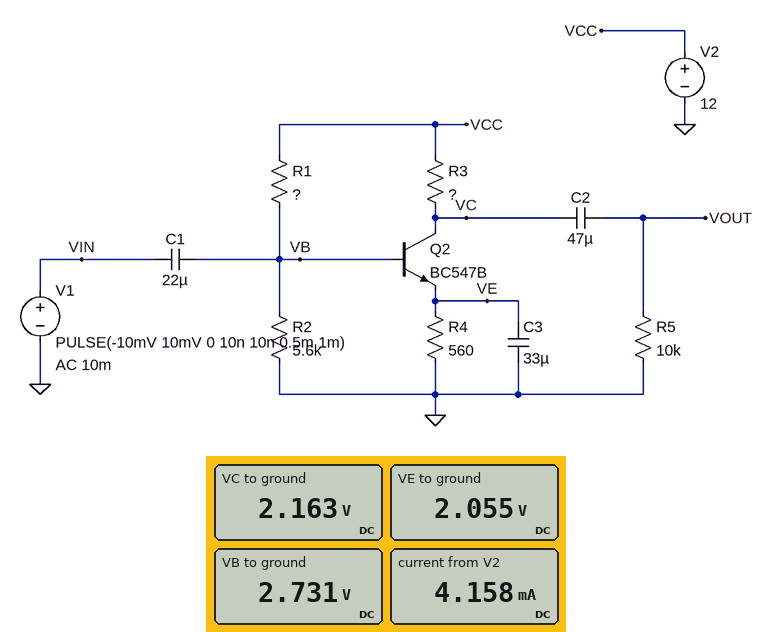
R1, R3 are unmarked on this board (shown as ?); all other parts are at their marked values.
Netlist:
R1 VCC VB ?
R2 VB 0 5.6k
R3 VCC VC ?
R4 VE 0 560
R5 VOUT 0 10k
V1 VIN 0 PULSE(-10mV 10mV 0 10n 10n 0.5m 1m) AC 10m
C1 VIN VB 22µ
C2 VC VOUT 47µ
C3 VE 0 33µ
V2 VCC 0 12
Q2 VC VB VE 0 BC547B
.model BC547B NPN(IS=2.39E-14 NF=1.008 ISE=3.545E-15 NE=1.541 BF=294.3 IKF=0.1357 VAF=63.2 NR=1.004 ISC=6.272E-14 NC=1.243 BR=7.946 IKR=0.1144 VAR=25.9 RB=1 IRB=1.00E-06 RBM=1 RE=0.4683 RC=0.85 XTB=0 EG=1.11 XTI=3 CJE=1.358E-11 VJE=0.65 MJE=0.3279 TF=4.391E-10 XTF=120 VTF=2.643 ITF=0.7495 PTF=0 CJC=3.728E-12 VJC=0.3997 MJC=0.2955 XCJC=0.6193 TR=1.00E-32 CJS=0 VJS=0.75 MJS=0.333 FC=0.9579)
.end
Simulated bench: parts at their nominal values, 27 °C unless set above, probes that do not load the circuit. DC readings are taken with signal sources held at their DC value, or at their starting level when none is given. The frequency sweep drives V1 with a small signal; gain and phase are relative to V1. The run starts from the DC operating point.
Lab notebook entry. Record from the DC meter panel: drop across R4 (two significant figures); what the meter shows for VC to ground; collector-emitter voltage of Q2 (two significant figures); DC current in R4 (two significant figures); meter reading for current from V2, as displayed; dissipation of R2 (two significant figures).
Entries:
2.1 V
2.163 V
110 mV
3.7 mA
4.158 mA
1.3 mW
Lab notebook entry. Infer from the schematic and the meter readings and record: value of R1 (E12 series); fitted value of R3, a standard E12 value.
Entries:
18 kΩ
2.7 kΩ
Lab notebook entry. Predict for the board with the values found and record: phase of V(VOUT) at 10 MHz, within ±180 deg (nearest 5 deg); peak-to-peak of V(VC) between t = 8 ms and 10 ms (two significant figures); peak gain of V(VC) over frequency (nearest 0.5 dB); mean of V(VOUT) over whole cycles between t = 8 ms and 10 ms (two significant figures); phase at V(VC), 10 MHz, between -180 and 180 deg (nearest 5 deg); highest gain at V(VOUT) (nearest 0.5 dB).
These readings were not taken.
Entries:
145 deg
2.8 V
30.0 dB
670 mV
145 deg
30.0 dB
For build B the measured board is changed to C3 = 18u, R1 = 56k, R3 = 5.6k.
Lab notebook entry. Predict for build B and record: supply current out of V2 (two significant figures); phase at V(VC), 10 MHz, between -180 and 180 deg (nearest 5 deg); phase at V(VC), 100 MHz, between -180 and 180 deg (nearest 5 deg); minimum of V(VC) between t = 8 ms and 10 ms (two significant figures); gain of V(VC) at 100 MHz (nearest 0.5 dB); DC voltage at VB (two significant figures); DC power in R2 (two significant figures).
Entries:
990 µA
160 deg
100 deg
5.9 V
29.0 dB
1.1 V
210 µW
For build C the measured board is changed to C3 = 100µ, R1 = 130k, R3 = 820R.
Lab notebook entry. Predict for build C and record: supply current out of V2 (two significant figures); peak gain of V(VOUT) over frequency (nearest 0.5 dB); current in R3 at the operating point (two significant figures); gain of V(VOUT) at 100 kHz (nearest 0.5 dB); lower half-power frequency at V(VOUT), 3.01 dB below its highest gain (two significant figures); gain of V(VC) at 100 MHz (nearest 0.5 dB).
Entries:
93 µA
0 dB
4.5 µA
-17.5 dB
140 MHz
-5.0 dB
